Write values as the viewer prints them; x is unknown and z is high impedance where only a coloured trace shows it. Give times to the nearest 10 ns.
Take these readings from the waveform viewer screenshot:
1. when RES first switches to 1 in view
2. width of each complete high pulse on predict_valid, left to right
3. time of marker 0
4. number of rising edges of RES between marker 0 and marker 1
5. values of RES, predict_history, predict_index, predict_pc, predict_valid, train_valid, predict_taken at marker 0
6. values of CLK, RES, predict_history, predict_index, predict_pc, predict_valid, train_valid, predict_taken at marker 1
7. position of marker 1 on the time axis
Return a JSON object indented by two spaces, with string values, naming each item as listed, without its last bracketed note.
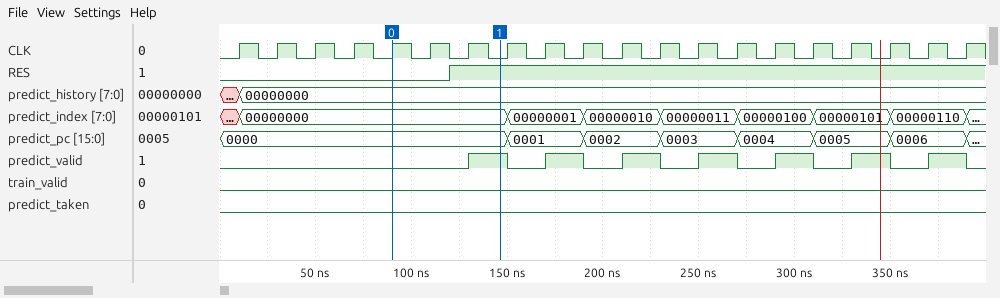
{
  "when RES first switches to 1 in view": "120 ns",
  "width of each complete high pulse on predict_valid, left to right": "20 ns, 20 ns, 20 ns, 20 ns, 20 ns, 20 ns, 20 ns",
  "time of marker 0": "90 ns",
  "number of rising edges of RES between marker 0 and marker 1": "1",
  "values of RES, predict_history, predict_index, predict_pc, predict_valid, train_valid, predict_taken at marker 0": "RES=0, predict_history=00000000, predict_index=00000000, predict_pc=0000, predict_valid=0, train_valid=0, predict_taken=0",
  "values of CLK, RES, predict_history, predict_index, predict_pc, predict_valid, train_valid, predict_taken at marker 1": "CLK=0, RES=1, predict_history=00000000, predict_index=00000000, predict_pc=0000, predict_valid=1, train_valid=0, predict_taken=0",
  "position of marker 1 on the time axis": "150 ns"
}
